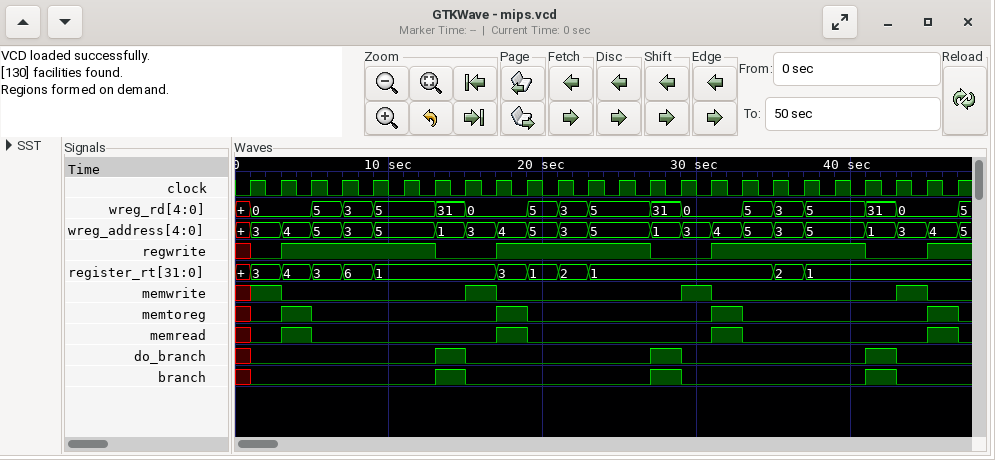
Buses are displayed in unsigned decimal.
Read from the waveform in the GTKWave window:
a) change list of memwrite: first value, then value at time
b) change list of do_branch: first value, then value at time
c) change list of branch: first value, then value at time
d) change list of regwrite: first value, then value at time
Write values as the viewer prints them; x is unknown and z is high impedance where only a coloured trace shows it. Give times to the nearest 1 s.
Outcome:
x, 1 at 1 s, 0 at 3 s, 1 at 15 s, 0 at 17 s, 1 at 29 s, 0 at 31 s, 1 at 43 s, 0 at 45 s
x, 0 at 1 s, 1 at 13 s, 0 at 15 s, 1 at 27 s, 0 at 29 s, 1 at 41 s, 0 at 43 s
x, 0 at 1 s, 1 at 13 s, 0 at 15 s, 1 at 27 s, 0 at 29 s, 1 at 41 s, 0 at 43 s
x, 0 at 1 s, 1 at 3 s, 0 at 13 s, 1 at 17 s, 0 at 27 s, 1 at 31 s, 0 at 41 s, 1 at 45 s
